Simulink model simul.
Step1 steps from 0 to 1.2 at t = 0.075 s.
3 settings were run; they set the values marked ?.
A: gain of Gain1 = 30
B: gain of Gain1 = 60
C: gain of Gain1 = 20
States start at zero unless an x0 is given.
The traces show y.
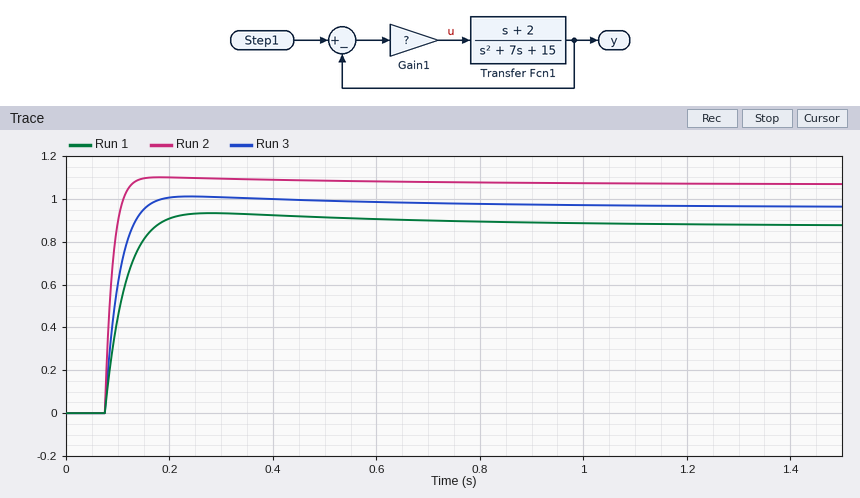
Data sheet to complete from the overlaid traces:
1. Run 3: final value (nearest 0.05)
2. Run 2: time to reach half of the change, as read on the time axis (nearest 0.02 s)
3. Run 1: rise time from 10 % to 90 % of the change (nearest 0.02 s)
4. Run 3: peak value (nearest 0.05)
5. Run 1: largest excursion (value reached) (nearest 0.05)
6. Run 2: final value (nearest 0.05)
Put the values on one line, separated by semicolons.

0.95; 0.08 s; 0.06 s; 1.00; 0.95; 1.05
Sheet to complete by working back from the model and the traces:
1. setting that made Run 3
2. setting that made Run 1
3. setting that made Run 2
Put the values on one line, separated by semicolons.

A; C; B
